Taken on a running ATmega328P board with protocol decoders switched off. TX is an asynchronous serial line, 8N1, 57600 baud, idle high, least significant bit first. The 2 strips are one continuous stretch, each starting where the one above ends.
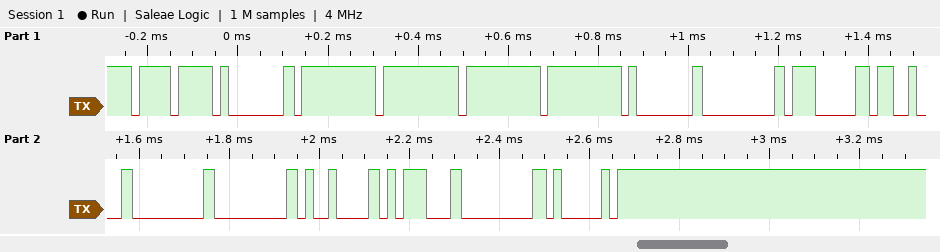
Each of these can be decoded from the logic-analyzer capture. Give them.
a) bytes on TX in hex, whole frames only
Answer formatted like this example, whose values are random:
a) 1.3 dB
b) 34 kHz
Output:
a) 0xEF 0x01 0xFF 0xFF 0xFF 0xFF 0x01 0x00 0x07 0x13 0x00 0x00 0x09 0x1D 0x00 0x41
